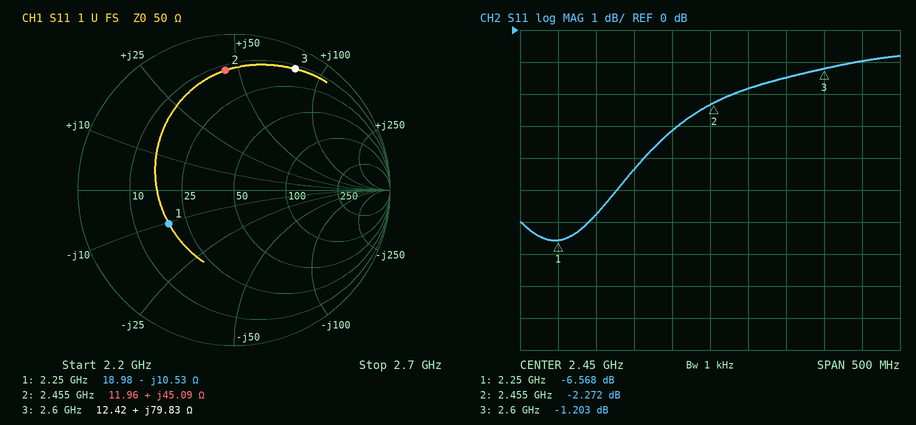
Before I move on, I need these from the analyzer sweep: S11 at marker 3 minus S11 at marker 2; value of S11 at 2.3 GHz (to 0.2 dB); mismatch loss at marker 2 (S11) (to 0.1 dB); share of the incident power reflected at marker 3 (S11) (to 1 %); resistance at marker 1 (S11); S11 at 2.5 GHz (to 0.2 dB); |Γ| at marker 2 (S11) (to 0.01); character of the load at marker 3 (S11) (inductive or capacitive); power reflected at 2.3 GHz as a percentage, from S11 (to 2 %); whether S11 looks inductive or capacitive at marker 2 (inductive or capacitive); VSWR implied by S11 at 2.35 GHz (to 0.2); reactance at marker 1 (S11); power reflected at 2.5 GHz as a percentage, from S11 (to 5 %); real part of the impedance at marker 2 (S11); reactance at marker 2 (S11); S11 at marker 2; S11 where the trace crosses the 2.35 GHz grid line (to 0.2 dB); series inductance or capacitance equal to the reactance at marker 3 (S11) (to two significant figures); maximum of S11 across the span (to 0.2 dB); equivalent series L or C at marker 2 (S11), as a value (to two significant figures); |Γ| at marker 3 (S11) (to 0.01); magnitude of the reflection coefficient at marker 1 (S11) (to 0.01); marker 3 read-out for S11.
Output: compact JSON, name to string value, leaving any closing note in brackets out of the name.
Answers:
{"S11 at marker 3 minus S11 at marker 2": "1.069 dB", "value of S11 at 2.3 GHz": "-5.8 dB", "mismatch loss at marker 2 (S11)": "3.9 dB", "share of the incident power reflected at marker 3 (S11)": "76 %", "resistance at marker 1": "18.98 Ω", "S11 at 2.5 GHz": "-1.8 dB", "|Γ| at marker 2 (S11)": "0.77", "character of the load at marker 3 (S11)": "inductive", "power reflected at 2.3 GHz as a percentage, from S11": "26 %", "whether S11 looks inductive or capacitive at marker 2": "inductive", "VSWR implied by S11 at 2.35 GHz": "4.0", "reactance at marker 1": "-10.53 Ω", "power reflected at 2.5 GHz as a percentage, from S11": "65 %", "real part of the impedance at marker 2": "11.96 Ω", "reactance at marker 2": "+45.09 Ω", "S11 at marker 2": "-2.272 dB", "S11 where the trace crosses the 2.35 GHz grid line": "-4.4 dB", "series inductance or capacitance equal to the reactance at marker 3 (S11)": "4.9 nH", "maximum of S11 across the span": "-0.8 dB", "equivalent series L or C at marker 2 (S11), as a value": "2.9 nH", "|Γ| at marker 3 (S11)": "0.87", "magnitude of the reflection coefficient at marker 1 (S11)": "0.47", "marker 3 read-out for S11": "-1.203 dB"}
